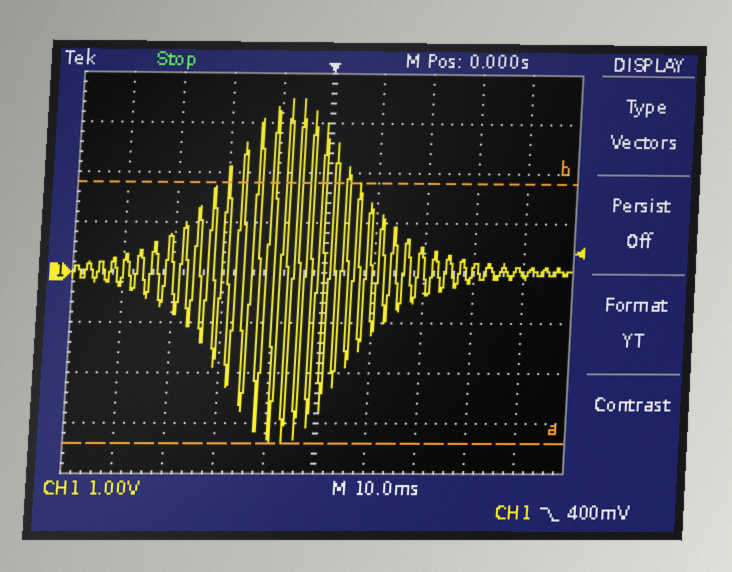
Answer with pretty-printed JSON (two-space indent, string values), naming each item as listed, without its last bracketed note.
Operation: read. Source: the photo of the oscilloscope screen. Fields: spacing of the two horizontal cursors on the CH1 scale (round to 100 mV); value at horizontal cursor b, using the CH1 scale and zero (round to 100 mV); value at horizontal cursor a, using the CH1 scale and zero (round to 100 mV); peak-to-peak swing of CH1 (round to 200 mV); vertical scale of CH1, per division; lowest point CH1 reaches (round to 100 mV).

{
  "spacing of the two horizontal cursors on the CH1 scale": "5.2 V",
  "value at horizontal cursor b, using the CH1 scale and zero": "1.8 V",
  "value at horizontal cursor a, using the CH1 scale and zero": "-3.4 V",
  "peak-to-peak swing of CH1": "6.8 V",
  "vertical scale of CH1, per division": "1 V",
  "lowest point CH1 reaches": "-3.4 V"
}
